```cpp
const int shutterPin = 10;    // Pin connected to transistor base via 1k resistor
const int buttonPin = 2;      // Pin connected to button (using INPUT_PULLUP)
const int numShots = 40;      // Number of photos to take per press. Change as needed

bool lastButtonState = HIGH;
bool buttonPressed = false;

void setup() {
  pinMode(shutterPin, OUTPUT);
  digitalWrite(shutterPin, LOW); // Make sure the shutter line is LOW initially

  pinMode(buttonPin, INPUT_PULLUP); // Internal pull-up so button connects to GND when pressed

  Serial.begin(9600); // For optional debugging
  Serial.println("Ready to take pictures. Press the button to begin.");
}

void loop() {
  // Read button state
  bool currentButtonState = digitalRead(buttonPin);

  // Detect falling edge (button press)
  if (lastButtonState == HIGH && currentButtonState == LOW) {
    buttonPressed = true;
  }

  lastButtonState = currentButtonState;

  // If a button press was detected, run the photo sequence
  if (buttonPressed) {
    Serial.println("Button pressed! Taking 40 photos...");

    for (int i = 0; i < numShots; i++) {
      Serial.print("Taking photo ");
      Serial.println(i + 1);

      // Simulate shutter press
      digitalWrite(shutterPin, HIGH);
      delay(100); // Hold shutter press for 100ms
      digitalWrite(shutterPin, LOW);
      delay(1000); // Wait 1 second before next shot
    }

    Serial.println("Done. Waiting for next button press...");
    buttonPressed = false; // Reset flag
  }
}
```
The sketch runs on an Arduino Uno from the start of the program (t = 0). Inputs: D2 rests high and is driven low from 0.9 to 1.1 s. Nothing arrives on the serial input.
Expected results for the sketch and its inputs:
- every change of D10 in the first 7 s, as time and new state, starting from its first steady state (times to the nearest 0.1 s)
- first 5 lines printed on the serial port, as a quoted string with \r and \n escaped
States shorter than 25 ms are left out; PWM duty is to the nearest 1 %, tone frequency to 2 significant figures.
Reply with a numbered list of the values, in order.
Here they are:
1. 0 s low; 0.9 s high; 1 s low; 2 s high; 2.1 s low; 3.1 s high; 3.2 s low; 4.2 s high; 4.3 s low; 5.3 s high; 5.4 s low; 6.4 s high; 6.5 s low
2. "Ready to take pictures. Press the button to begin.\r\nButton pressed! Taking 40 photos...\r\nTaking photo 1\r\nTaking photo 2\r\nTaking photo 3\r\n"
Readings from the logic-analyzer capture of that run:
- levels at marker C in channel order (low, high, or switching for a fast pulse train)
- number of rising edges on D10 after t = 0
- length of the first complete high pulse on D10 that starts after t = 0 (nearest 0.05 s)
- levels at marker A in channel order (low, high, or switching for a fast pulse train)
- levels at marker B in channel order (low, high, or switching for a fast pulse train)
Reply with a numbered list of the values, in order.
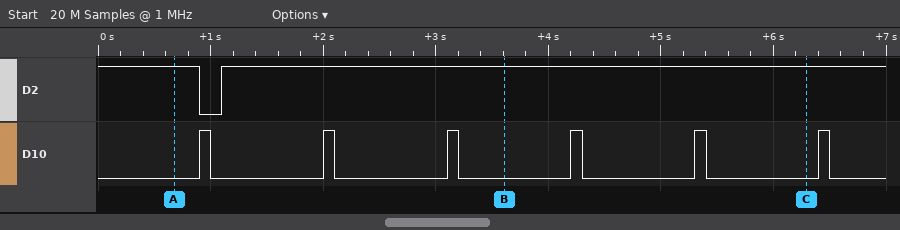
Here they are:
1. D2 high, D10 low
2. 6
3. 0.10 s
4. D2 high, D10 low
5. D2 high, D10 low
